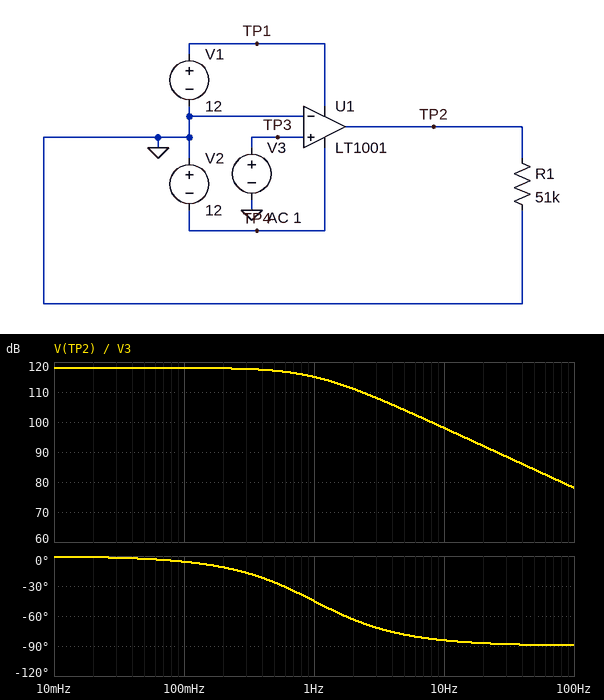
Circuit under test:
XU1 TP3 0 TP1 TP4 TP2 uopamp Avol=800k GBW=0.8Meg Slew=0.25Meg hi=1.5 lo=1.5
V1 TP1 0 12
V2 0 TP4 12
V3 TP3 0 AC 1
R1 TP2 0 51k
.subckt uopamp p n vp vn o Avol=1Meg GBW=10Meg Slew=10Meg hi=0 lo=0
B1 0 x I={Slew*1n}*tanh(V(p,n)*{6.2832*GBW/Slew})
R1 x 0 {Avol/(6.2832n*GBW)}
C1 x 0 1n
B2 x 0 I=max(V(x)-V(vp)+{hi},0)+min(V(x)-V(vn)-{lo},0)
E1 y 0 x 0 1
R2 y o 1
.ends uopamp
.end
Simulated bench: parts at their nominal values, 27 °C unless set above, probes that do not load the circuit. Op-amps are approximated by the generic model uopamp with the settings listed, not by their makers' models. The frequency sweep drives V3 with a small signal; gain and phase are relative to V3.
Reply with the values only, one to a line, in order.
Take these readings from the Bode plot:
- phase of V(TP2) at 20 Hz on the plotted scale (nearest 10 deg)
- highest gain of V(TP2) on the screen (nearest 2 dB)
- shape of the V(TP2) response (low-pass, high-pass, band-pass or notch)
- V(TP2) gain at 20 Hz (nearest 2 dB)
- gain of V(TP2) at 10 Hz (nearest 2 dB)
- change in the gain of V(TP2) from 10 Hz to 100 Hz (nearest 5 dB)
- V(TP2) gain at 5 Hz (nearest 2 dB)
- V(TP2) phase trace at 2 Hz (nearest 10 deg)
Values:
-90 deg
118 dB
low-pass
92 dB
98 dB
-20 dB
104 dB
-60 deg
